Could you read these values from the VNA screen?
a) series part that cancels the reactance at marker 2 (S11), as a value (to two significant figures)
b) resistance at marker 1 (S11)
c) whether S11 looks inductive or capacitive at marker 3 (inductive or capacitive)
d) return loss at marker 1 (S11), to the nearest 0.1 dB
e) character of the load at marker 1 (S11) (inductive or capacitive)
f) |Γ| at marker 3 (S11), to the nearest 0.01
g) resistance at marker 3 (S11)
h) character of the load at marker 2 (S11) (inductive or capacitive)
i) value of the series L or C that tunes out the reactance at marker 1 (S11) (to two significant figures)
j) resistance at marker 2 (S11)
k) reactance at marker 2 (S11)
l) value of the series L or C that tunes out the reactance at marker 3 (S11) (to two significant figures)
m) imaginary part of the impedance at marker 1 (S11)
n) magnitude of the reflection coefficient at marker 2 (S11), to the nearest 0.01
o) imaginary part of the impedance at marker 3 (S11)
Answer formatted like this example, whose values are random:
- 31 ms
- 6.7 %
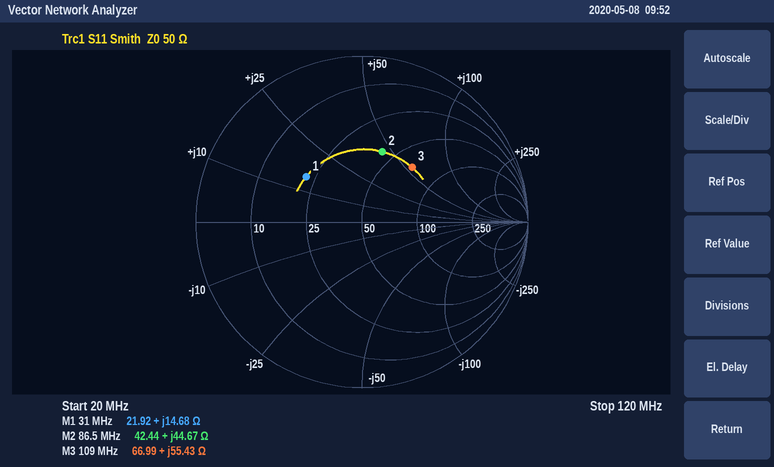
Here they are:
- 41 pF
- 21.92 Ω
- inductive
- 7.3 dB
- inductive
- 0.45
- 66.99 Ω
- inductive
- 350 pF
- 42.44 Ω
- +44.67 Ω
- 26 pF
- +14.68 Ω
- 0.44
- +55.43 Ω
